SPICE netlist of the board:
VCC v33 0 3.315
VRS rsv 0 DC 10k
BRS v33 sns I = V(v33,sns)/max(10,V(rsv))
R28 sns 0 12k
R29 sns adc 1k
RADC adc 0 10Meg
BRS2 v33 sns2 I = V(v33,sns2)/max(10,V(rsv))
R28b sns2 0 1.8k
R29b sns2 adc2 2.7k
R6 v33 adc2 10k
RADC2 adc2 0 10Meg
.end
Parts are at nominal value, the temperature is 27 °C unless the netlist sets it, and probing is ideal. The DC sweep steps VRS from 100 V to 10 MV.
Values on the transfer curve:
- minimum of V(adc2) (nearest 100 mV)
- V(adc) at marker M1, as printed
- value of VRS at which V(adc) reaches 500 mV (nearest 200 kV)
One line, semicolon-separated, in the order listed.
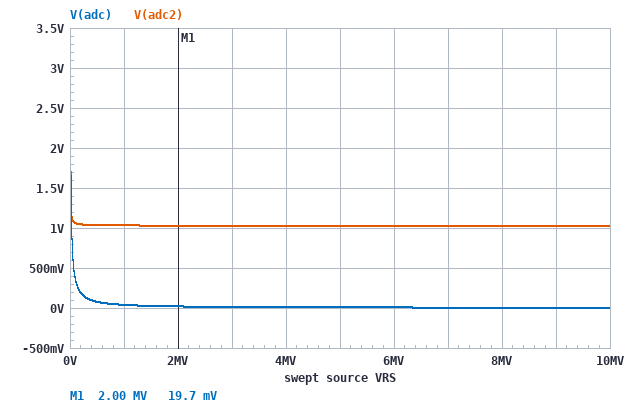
1.0 V; 19.7 mV; 0 V
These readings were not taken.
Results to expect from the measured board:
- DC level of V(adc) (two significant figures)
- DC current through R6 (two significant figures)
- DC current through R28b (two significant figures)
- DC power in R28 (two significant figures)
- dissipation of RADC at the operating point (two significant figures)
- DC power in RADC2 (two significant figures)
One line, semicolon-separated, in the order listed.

1.8 V; 200 µA; 450 µA; 270 µW; 330 nW; 180 nW
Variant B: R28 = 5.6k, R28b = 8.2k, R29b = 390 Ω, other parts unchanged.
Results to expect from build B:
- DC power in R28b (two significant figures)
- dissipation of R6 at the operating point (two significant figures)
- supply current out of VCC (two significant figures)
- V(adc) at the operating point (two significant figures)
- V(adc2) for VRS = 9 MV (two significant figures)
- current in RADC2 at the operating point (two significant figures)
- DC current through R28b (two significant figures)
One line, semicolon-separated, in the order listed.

510 µW; 150 µW; 460 µA; 1.2 V; 1.5 V; 210 nA; 250 µA
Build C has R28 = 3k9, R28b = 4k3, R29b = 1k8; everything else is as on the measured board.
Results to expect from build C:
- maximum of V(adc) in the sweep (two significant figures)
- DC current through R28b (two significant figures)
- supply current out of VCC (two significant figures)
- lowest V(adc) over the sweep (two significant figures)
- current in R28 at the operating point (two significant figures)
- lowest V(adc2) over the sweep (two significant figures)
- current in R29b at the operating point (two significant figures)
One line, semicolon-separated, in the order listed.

3.2 V; 340 µA; 580 µA; 1.3 mV; 240 µA; 1.3 V; 160 µA
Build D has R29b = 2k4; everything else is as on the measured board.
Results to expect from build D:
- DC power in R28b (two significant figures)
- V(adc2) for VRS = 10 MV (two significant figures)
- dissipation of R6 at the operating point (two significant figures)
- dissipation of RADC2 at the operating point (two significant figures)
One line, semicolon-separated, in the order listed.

370 µW; 980 mV; 410 µW; 170 nW
